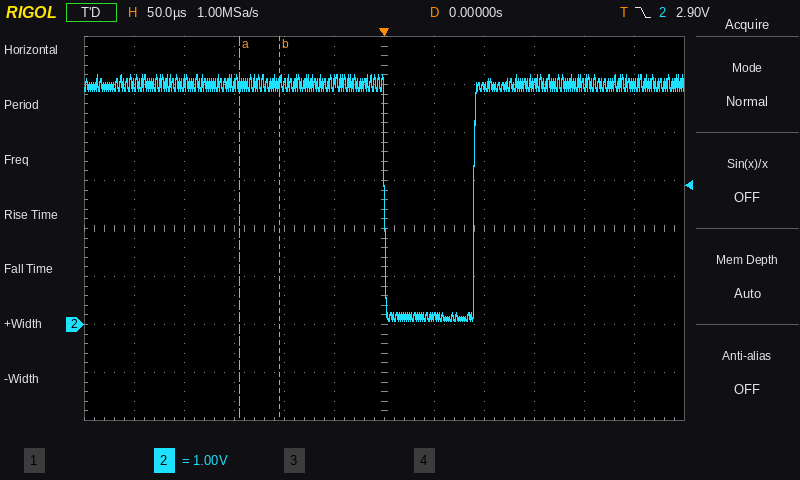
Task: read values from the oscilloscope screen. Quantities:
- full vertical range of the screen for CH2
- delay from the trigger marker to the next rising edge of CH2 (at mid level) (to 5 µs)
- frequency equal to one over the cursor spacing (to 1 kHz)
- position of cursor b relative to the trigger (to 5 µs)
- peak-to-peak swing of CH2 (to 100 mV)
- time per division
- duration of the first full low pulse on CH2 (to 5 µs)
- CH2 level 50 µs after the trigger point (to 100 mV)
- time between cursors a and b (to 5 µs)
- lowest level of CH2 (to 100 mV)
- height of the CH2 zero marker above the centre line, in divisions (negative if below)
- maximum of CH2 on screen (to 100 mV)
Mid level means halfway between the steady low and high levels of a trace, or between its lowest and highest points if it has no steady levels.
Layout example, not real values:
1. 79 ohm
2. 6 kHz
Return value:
1. 8 V
2. 90 µs
3. 25 kHz
4. -105 µs
5. 5.1 V
6. 50 µs
7. 90 µs
8. 200 mV
9. 40 µs
10. 100 mV
11. -2.0 div
12. 5.2 V
